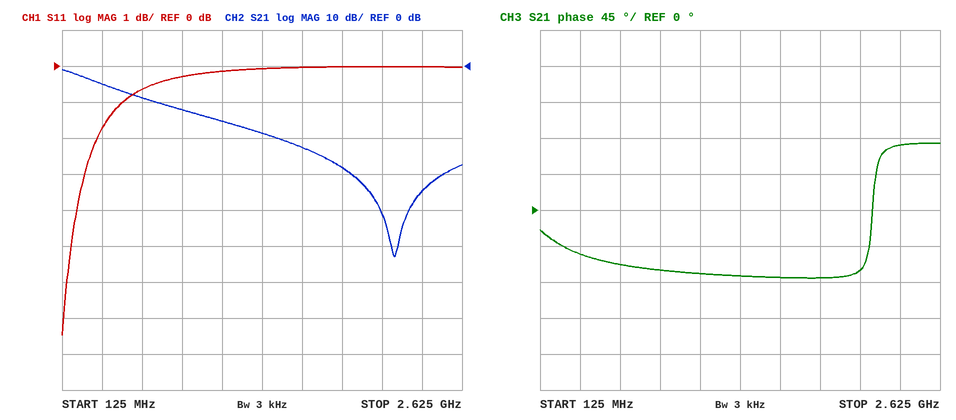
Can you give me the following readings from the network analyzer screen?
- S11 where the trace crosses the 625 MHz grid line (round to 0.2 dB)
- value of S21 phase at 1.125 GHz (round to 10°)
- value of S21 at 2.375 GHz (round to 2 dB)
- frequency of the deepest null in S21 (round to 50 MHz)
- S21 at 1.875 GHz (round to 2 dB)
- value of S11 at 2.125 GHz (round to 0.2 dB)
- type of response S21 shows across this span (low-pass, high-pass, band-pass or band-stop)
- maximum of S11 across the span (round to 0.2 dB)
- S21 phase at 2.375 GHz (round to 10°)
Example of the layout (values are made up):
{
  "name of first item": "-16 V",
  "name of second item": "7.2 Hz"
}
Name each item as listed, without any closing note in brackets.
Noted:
{
  "S11 where the trace crosses the 625 MHz grid line": "-0.6 dB",
  "value of S21 phase at 1.125 GHz": "-80°",
  "value of S21 at 2.375 GHz": "-34 dB",
  "frequency of the deepest null in S21": "2.20 GHz",
  "S21 at 1.875 GHz": "-28 dB",
  "value of S11 at 2.125 GHz": "0.0 dB",
  "type of response S21 shows across this span": "low-pass",
  "maximum of S11 across the span": "0.0 dB",
  "S21 phase at 2.375 GHz": "80°"
}
